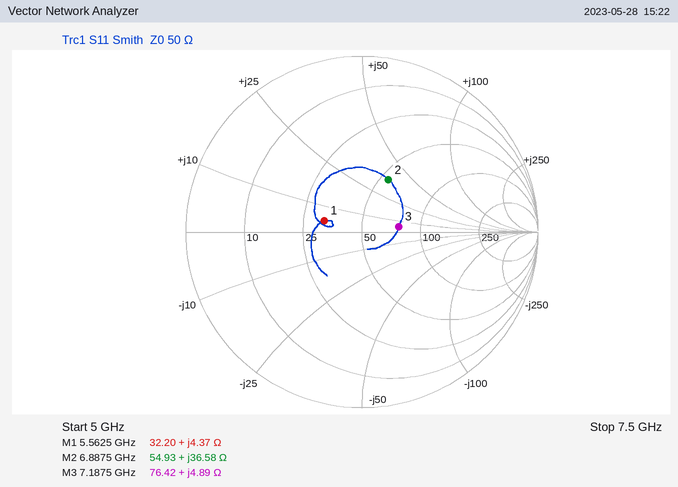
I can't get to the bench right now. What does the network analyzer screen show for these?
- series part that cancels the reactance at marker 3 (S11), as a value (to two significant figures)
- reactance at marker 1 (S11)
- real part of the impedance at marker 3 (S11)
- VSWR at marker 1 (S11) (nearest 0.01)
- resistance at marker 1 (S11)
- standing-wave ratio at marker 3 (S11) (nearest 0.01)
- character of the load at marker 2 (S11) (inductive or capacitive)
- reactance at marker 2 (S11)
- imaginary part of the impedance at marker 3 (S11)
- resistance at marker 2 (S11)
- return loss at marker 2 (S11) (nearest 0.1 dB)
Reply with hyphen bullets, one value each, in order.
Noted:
- 4.5 pF
- +4.37 Ω
- 76.42 Ω
- 1.57
- 32.20 Ω
- 1.54
- inductive
- +36.58 Ω
- +4.89 Ω
- 54.93 Ω
- 9.6 dB
